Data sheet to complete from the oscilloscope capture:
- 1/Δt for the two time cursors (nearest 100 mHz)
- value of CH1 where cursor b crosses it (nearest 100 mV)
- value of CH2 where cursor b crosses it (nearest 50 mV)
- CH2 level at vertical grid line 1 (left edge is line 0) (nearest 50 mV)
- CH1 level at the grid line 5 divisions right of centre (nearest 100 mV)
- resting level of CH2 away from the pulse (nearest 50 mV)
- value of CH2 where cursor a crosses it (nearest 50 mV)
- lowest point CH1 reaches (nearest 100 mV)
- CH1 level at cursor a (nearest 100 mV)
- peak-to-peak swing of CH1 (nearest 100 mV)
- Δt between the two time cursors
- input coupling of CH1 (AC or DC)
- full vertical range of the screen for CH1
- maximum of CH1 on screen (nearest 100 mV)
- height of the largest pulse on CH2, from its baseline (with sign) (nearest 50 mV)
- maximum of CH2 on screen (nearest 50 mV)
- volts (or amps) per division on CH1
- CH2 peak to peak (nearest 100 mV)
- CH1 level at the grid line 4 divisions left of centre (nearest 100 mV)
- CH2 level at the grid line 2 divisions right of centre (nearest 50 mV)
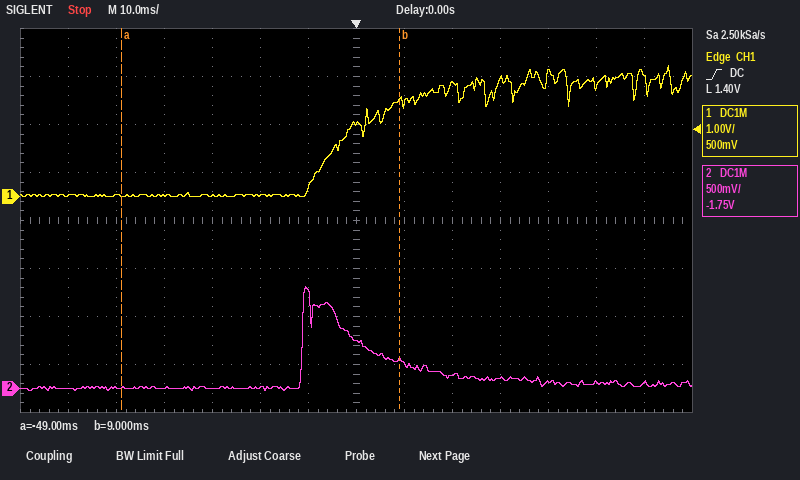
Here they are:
17.2 Hz
2.0 V
300 mV
0 mV
2.3 V
0 mV
0 mV
0.0 V
0.0 V
2.7 V
58 ms
DC
8 V
2.7 V
+1.05 V
1.05 V
1 V
1.10 V
0.0 V
150 mV
